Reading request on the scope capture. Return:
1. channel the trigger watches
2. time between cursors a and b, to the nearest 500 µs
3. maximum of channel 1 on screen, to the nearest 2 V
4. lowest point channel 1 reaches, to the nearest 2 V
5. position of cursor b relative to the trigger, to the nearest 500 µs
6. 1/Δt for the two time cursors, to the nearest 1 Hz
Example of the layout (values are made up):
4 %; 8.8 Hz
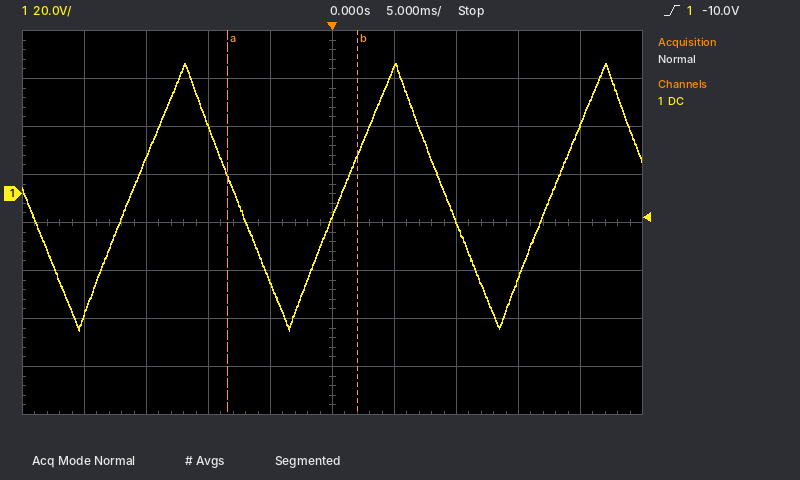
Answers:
channel 1; 10.5 ms; 54 V; -56 V; +2.0 ms; 95 Hz
